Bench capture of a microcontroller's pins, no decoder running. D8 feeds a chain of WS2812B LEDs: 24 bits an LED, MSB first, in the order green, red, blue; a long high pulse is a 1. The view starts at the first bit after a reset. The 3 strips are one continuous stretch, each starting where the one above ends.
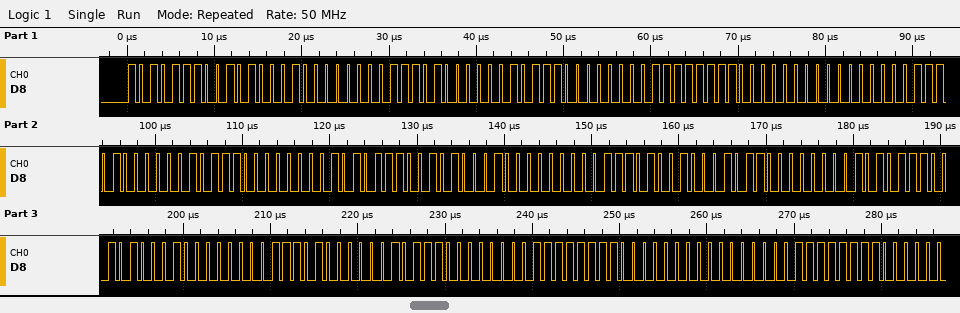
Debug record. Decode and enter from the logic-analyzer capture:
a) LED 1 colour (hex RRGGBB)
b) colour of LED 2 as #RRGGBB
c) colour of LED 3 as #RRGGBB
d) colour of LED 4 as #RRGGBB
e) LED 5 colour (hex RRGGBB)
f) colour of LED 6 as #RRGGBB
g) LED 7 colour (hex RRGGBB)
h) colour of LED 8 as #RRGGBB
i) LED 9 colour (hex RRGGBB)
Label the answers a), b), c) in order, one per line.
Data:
a) #51AE00
b) #17E800
c) #00FF00
d) #17E800
e) #51AE00
f) #8B7400
g) #51AE00
h) #17E800
i) #00FF00
